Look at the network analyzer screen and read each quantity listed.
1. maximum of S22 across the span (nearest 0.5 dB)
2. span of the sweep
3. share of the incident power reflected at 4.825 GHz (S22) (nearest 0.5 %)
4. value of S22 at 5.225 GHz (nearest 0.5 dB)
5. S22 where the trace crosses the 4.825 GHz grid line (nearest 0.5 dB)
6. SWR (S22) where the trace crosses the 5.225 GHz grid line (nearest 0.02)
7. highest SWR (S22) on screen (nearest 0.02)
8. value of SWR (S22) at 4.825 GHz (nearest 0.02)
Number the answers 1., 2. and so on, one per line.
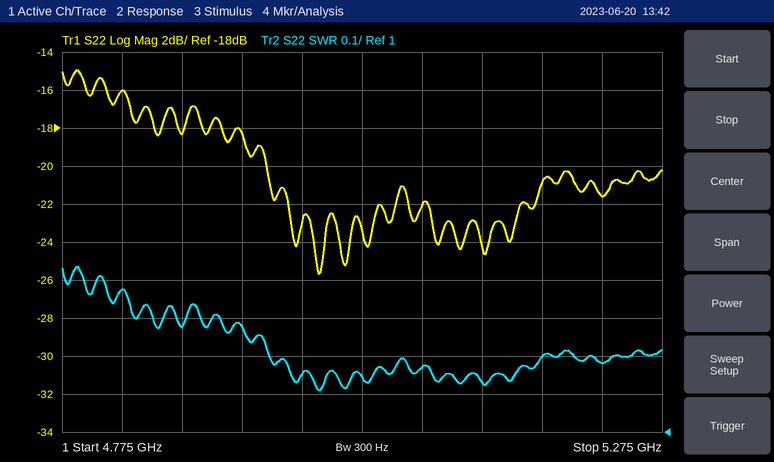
1. -15.0 dB
2. 500 MHz
3. 2.5 %
4. -21.5 dB
5. -16.0 dB
6. 1.18
7. 1.44
8. 1.38
